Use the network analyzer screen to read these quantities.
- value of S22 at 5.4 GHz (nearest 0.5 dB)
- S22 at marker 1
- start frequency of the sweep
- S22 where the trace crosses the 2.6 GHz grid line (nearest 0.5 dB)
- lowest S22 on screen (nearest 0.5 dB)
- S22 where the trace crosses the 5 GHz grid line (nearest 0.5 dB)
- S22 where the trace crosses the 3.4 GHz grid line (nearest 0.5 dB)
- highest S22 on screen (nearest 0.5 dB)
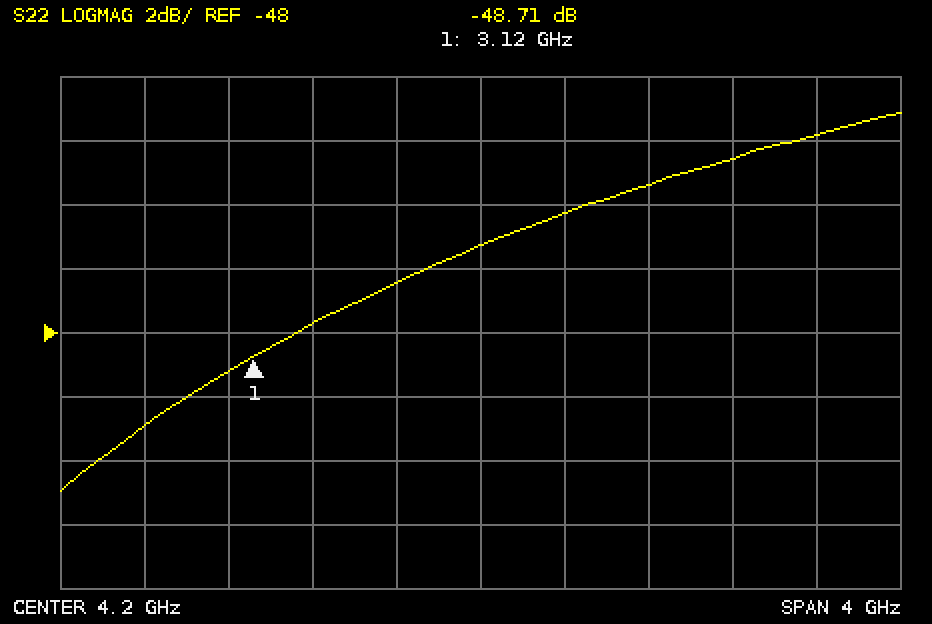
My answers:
-42.5 dB
-48.71 dB
2.2 GHz
-51.0 dB
-53.0 dB
-43.5 dB
-47.5 dB
-41.0 dB
